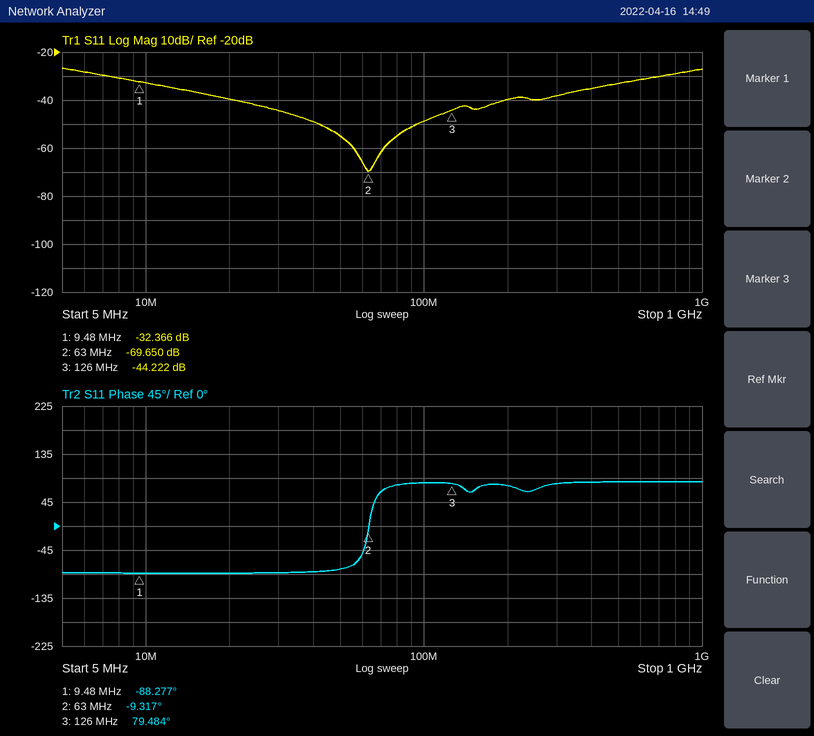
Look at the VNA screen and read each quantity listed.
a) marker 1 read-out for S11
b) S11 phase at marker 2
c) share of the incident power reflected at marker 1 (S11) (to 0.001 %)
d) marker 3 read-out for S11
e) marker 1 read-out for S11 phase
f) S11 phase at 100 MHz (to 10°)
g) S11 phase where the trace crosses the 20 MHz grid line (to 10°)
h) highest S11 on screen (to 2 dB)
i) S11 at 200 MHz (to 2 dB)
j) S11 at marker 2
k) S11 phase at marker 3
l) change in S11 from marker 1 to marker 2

-32.366 dB
-9.317°
0.058 %
-44.222 dB
-88.277°
80°
-90°
-26 dB
-40 dB
-69.650 dB
79.484°
-37.284 dB
